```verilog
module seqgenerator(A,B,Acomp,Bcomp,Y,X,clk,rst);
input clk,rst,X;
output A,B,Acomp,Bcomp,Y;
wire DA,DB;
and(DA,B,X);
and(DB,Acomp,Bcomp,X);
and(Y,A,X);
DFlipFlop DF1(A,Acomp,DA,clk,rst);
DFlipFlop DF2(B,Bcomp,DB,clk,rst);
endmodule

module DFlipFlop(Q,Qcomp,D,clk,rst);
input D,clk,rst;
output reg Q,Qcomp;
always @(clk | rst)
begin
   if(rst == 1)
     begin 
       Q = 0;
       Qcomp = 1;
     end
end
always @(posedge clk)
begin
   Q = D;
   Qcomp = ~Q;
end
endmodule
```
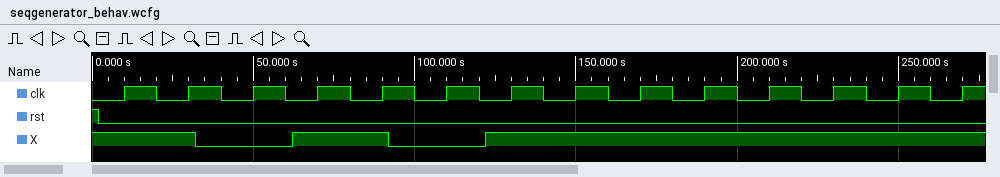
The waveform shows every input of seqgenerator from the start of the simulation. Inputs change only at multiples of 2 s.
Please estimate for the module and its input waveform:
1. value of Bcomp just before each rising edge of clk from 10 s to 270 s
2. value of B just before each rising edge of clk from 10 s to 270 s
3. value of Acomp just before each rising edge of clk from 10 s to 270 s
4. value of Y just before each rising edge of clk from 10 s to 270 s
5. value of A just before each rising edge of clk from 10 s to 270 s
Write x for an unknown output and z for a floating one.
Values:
1 0 1 1 0 1 1 0 1 1 0 1 1 0
0 1 0 0 1 0 0 1 0 0 1 0 0 1
1 1 0 1 1 0 1 1 0 1 1 0 1 1
0 0 0 0 0 0 0 0 1 0 0 1 0 0
0 0 1 0 0 1 0 0 1 0 0 1 0 0
